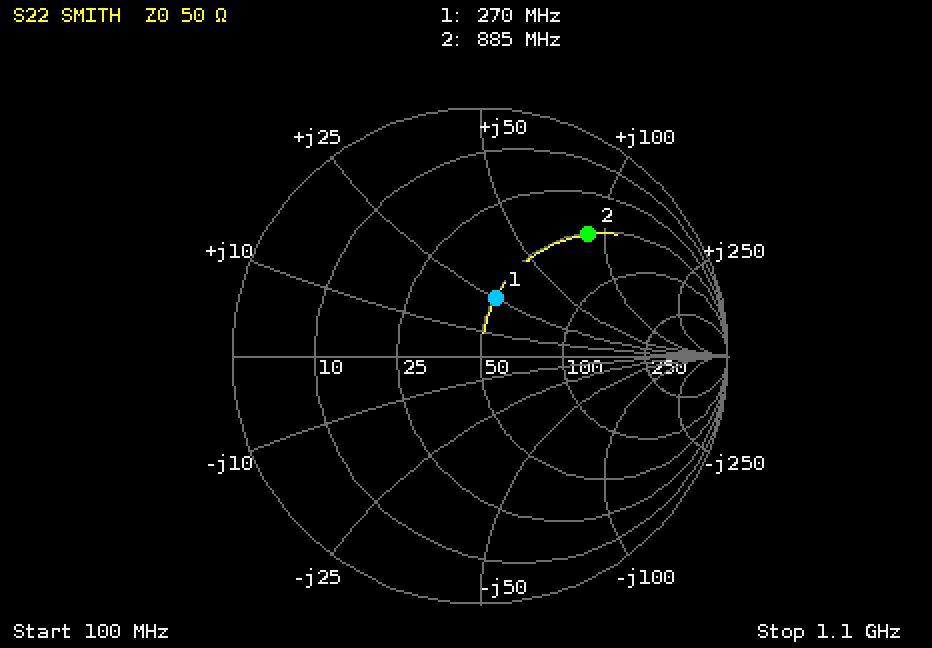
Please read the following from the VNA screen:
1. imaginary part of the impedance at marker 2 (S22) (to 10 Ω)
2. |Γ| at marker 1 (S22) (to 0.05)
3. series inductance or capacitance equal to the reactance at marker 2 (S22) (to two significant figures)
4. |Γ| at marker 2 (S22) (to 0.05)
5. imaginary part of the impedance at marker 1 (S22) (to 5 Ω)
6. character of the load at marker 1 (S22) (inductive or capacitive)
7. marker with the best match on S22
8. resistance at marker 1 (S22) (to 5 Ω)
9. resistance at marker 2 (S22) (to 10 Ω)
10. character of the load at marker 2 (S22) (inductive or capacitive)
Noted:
+90 Ω
0.25
16 nH
0.65
+25 Ω
inductive
marker 1
50 Ω
50 Ω
inductive
